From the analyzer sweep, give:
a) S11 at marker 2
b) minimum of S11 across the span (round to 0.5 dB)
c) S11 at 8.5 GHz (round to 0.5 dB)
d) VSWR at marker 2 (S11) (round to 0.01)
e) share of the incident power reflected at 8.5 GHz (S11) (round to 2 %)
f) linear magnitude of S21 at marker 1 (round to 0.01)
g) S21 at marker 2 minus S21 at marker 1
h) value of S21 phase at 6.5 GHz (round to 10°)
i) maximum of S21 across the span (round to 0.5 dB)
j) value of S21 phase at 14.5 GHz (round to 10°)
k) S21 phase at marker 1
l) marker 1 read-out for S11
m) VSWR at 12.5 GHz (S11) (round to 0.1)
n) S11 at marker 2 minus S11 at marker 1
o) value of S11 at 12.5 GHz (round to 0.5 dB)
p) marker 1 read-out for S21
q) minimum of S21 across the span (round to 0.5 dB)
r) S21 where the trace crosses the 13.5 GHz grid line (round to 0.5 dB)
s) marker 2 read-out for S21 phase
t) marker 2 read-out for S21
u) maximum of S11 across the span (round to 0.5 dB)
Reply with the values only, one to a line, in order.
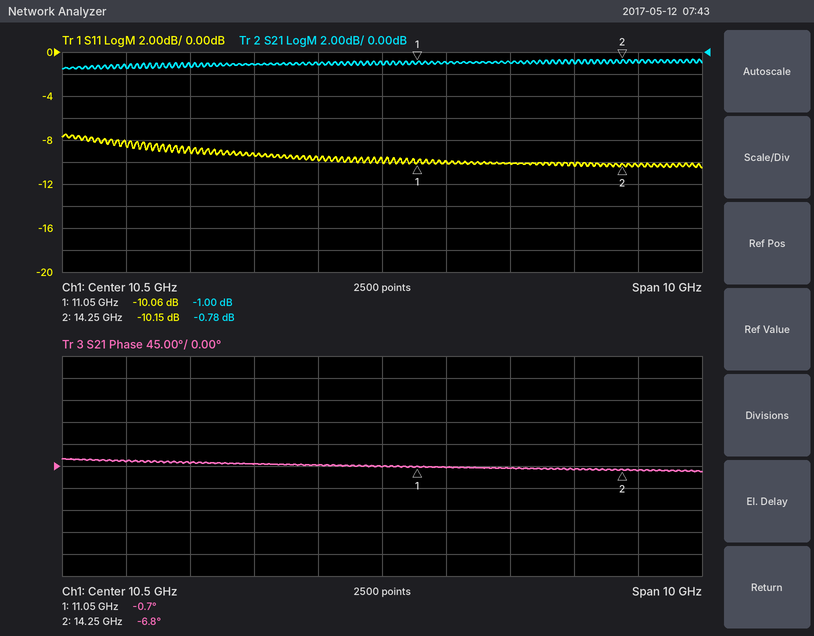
-10.15 dB
-10.5 dB
-9.5 dB
1.90
12 %
0.89
0.22 dB
10°
-0.5 dB
-10°
-0.7°
-10.06 dB
1.9
-0.09 dB
-10.0 dB
-1.00 dB
-1.5 dB
-1.0 dB
-6.8°
-0.78 dB
-7.5 dB
